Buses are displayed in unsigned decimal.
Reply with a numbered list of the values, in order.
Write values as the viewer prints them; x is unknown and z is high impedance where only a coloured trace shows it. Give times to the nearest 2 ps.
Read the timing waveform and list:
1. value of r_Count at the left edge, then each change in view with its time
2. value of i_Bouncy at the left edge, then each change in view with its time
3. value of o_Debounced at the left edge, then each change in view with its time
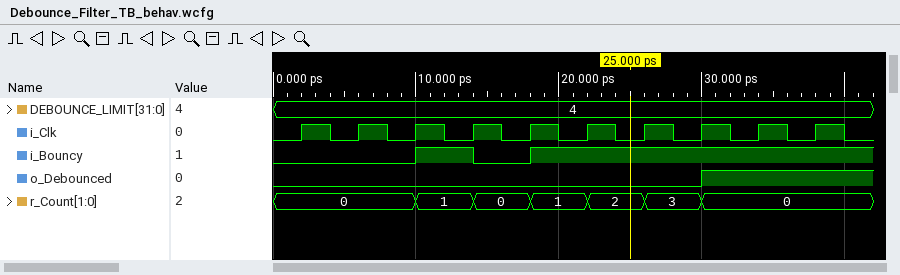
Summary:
1. 0, 1 at 10 ps, 0 at 14 ps, 1 at 18 ps, 2 at 22 ps, 3 at 26 ps, 0 at 30 ps
2. 0, 1 at 10 ps, 0 at 14 ps, 1 at 18 ps
3. 0, 1 at 30 ps
